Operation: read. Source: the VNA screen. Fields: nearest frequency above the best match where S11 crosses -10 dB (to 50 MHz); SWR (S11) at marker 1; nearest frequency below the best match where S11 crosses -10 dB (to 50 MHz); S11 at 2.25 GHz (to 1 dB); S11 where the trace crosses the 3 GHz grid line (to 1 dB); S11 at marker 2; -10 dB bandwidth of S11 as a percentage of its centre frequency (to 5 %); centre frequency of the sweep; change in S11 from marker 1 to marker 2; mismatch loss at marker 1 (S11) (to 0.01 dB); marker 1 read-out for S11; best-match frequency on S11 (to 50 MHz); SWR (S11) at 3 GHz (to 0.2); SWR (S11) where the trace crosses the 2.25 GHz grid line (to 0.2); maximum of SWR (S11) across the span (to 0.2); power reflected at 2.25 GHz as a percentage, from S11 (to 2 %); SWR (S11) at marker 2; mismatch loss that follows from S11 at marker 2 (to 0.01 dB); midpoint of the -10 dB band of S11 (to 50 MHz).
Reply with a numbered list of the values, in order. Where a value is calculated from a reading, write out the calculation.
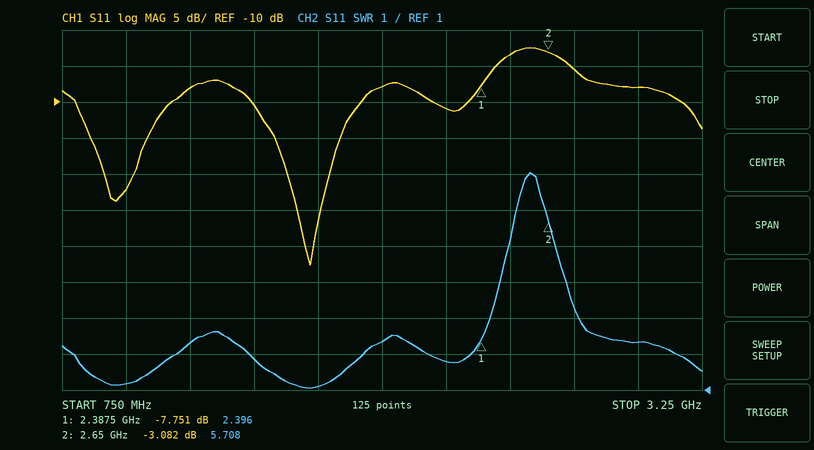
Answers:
1. 1.90 GHz
2. 2.396
3. 1.50 GHz
4. -11 dB
5. -8 dB
6. -3.082 dB
7. 400 MHz / 1.7 GHz ≈ 23.5 %, so 25 % to the nearest 5 %
8. 2 GHz
9. -3.082 − (-7.751) = 4.669 dB
10. −10 log10(1 − 10^(-7.751/10)) ≈ 0.80 dB
11. -7.751 dB
12. 1.70 GHz
13. 2.4
14. 1.8
15. 7.0
16. 10^(-11/10) ≈ 8 %
17. 5.708
18. −10 log10(1 − 10^(-3.082/10)) ≈ 2.94 dB
19. 1.70 GHz
